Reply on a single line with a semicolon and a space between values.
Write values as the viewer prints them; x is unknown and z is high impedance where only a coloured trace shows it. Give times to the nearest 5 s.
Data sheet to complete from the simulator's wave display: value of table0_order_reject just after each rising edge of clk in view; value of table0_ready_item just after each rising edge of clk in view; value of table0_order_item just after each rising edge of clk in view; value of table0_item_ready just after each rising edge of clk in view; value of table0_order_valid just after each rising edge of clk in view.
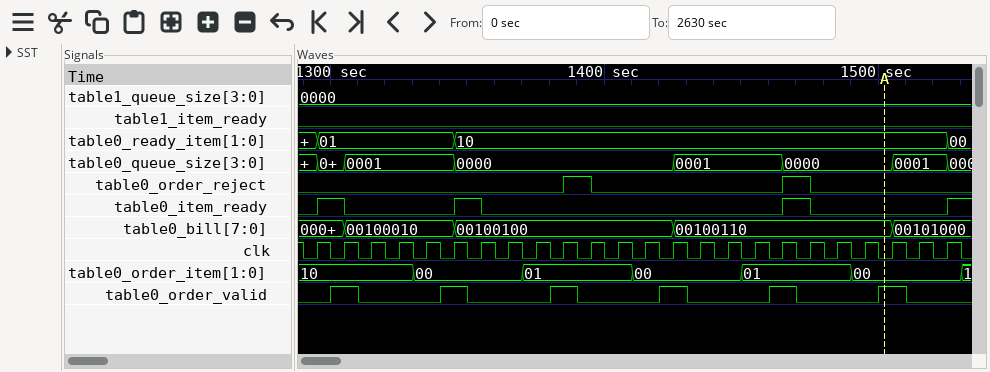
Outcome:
0 0 0 0 0 0 0 0 0 1 0 0 0 0 0 0 0 1 0 0 0 0 0 0; 01, 01, 01, 01, 01, 10, 10, 10, 10, 10, 10, 10, 10, 10, 10, 10, 10, 10, 10, 10, 10, 10, 10, 00; 10, 10, 10, 10, 00, 00, 00, 00, 01, 01, 01, 01, 00, 00, 00, 00, 01, 01, 01, 01, 00, 00, 00, 00; 1 0 0 0 0 1 0 0 0 0 0 0 0 0 0 0 0 1 0 0 0 0 0 1; 0 1 0 0 0 1 0 0 0 1 0 0 0 1 0 0 0 1 0 0 0 1 0 0
